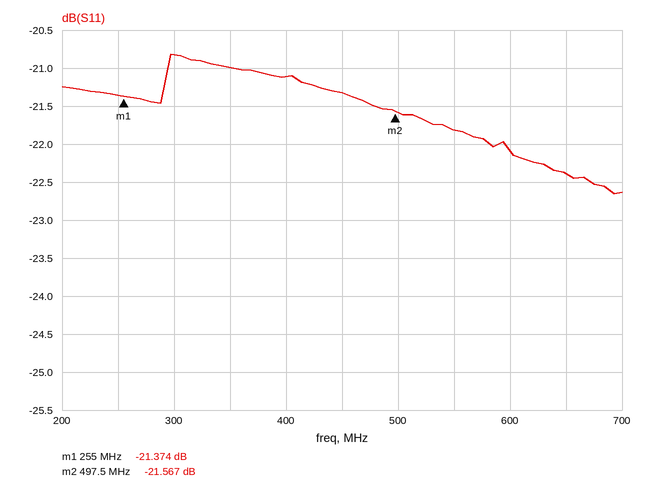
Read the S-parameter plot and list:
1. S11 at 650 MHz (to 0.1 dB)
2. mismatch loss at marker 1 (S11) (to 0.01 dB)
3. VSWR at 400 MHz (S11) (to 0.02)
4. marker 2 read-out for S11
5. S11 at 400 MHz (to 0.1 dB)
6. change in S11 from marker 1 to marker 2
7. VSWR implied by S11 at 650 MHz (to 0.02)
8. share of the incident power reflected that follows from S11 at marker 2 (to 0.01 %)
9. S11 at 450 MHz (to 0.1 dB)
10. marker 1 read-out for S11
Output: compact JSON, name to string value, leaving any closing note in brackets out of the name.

{"S11 at 650 MHz": "-22.4 dB", "mismatch loss at marker 1 (S11)": "0.03 dB", "VSWR at 400 MHz (S11)": "1.20", "marker 2 read-out for S11": "-21.567 dB", "S11 at 400 MHz": "-21.1 dB", "change in S11 from marker 1 to marker 2": "-0.193 dB", "VSWR implied by S11 at 650 MHz": "1.16", "share of the incident power reflected that follows from S11 at marker 2": "0.70 %", "S11 at 450 MHz": "-21.3 dB", "marker 1 read-out for S11": "-21.374 dB"}
